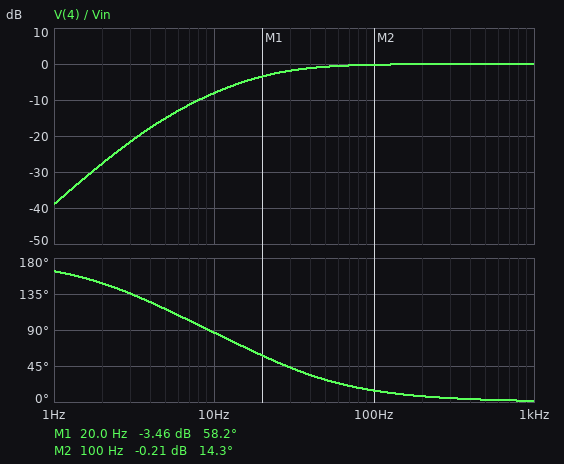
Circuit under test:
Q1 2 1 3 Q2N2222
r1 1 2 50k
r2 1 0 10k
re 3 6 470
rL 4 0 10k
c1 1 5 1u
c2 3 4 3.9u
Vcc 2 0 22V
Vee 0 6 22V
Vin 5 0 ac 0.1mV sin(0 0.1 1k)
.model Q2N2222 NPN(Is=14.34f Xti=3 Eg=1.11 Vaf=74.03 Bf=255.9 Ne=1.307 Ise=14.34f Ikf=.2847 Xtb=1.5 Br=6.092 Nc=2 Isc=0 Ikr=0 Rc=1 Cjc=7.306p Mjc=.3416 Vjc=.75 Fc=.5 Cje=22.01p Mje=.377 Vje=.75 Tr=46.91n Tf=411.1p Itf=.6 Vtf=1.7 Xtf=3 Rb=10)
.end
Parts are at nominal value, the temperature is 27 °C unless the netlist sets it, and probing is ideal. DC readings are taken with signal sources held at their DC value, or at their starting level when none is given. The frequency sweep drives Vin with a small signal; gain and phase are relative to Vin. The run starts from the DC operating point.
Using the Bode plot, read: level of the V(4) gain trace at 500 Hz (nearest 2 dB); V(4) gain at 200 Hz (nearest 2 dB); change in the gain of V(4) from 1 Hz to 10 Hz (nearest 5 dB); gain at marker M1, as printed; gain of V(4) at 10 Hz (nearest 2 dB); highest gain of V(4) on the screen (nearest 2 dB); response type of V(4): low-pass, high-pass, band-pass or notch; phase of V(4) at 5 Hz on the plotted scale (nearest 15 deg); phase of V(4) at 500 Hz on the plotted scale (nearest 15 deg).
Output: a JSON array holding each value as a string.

["0 dB", "0 dB", "30 dB", "-3.46 dB", "-8 dB", "0 dB", "high-pass", "120 deg", "0 deg"]
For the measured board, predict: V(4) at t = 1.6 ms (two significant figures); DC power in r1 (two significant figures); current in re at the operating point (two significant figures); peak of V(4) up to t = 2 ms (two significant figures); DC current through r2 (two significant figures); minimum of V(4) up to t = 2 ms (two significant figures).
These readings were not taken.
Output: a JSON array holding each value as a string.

["-63 mV", "8.1 mW", "49 mA", "98 mV", "180 µA", "-100 mV"]
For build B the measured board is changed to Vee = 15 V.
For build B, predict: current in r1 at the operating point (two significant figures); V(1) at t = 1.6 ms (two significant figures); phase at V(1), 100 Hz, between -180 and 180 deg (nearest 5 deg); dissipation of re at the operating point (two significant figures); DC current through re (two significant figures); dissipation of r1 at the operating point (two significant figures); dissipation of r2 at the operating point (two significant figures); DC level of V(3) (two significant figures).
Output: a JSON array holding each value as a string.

["390 µA", "2.3 V", "10 deg", "590 mW", "35 mA", "7.7 mW", "550 µW", "1.6 V"]
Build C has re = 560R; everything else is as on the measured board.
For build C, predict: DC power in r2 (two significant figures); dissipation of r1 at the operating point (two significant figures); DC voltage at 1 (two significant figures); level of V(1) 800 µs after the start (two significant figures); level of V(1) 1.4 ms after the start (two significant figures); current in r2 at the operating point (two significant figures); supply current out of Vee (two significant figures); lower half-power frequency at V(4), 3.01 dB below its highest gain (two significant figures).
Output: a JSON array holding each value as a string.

["440 µW", "7.9 mW", "2.1 V", "2.0 V", "2.2 V", "210 µA", "42 mA", "22 Hz"]
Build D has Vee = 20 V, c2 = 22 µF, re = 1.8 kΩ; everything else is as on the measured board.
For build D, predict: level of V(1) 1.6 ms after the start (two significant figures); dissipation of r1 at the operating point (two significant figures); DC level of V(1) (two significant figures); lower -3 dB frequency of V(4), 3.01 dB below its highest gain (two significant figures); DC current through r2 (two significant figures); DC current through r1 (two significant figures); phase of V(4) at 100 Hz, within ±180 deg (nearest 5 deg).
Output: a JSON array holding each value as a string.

["3.1 V", "7.1 mW", "3.2 V", "20 Hz", "320 µA", "380 µA", "10 deg"]
